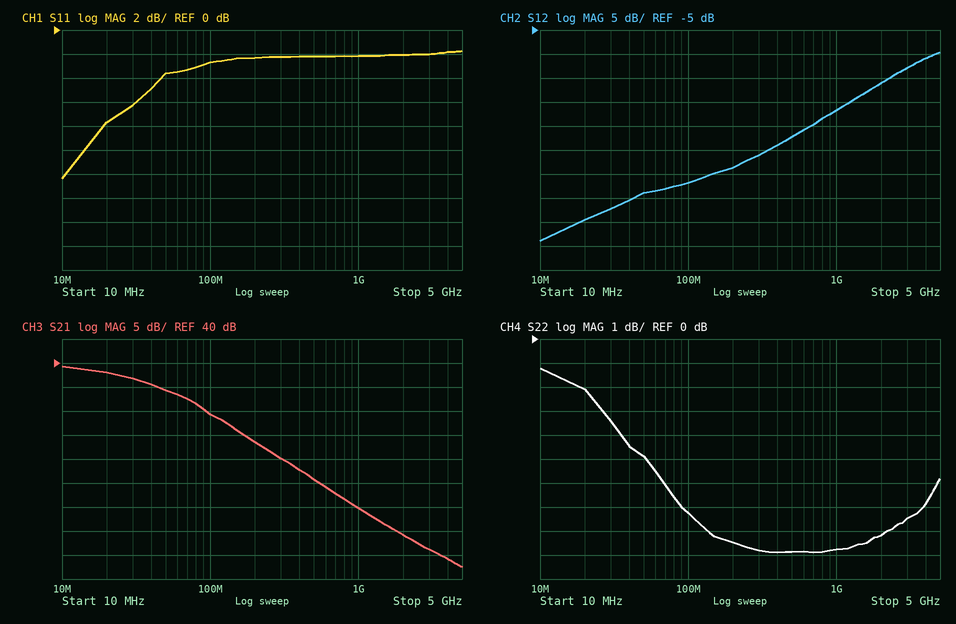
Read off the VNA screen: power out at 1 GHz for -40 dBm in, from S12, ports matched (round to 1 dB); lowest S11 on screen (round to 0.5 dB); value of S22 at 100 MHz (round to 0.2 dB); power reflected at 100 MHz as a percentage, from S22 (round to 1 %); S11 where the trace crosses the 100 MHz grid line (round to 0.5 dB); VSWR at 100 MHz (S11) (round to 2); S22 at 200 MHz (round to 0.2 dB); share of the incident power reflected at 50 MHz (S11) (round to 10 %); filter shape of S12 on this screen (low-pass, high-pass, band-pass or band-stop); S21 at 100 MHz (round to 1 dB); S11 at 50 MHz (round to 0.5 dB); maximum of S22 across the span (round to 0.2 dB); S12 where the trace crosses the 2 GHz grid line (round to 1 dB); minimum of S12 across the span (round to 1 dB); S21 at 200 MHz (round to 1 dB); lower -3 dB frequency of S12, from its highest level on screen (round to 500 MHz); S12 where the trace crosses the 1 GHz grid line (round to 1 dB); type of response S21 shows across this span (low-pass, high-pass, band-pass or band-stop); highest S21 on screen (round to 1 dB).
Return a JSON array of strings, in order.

["-62 dBm", "-12.5 dB", "-7.2 dB", "19 %", "-2.5 dB", "6", "-8.4 dB", "40 %", "high-pass", "29 dB", "-3.5 dB", "-1.2 dB", "-16 dB", "-49 dB", "24 dB", "3.0 GHz", "-22 dB", "low-pass", "39 dB"]
